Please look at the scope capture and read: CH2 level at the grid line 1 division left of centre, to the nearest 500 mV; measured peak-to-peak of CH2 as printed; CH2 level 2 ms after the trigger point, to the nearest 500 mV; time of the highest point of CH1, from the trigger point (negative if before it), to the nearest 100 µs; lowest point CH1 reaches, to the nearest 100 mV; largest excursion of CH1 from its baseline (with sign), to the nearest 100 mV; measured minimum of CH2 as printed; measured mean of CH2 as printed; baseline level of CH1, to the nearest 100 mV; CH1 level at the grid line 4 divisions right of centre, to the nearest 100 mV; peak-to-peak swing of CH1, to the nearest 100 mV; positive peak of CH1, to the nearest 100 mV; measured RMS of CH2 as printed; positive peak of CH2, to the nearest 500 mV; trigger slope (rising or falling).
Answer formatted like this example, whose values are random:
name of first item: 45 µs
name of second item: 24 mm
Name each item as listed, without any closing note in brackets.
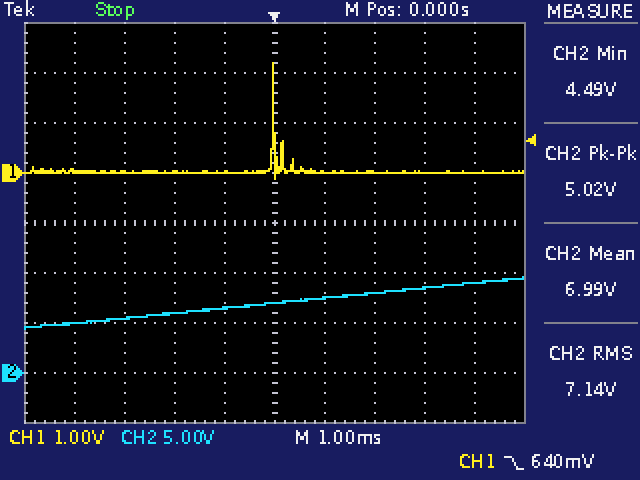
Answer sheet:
CH2 level at the grid line 1 division left of centre, to the nearest 500 mV: 6.5 V
measured peak-to-peak of CH2 as printed: 5.02 V
CH2 level 2 ms after the trigger point, to the nearest 500 mV: 8.0 V
time of the highest point of CH1, from the trigger point (negative if before it), to the nearest 100 µs: 0.0 ms
lowest point CH1 reaches, to the nearest 100 mV: -100 mV
largest excursion of CH1 from its baseline (with sign), to the nearest 100 mV: +2.2 V
measured minimum of CH2 as printed: 4.49 V
measured mean of CH2 as printed: 6.99 V
baseline level of CH1, to the nearest 100 mV: 0.0 V
CH1 level at the grid line 4 divisions right of centre, to the nearest 100 mV: 0.0 V
peak-to-peak swing of CH1, to the nearest 100 mV: 2.3 V
positive peak of CH1, to the nearest 100 mV: 2.2 V
measured RMS of CH2 as printed: 7.14 V
positive peak of CH2, to the nearest 500 mV: 9.5 V
trigger slope: falling
